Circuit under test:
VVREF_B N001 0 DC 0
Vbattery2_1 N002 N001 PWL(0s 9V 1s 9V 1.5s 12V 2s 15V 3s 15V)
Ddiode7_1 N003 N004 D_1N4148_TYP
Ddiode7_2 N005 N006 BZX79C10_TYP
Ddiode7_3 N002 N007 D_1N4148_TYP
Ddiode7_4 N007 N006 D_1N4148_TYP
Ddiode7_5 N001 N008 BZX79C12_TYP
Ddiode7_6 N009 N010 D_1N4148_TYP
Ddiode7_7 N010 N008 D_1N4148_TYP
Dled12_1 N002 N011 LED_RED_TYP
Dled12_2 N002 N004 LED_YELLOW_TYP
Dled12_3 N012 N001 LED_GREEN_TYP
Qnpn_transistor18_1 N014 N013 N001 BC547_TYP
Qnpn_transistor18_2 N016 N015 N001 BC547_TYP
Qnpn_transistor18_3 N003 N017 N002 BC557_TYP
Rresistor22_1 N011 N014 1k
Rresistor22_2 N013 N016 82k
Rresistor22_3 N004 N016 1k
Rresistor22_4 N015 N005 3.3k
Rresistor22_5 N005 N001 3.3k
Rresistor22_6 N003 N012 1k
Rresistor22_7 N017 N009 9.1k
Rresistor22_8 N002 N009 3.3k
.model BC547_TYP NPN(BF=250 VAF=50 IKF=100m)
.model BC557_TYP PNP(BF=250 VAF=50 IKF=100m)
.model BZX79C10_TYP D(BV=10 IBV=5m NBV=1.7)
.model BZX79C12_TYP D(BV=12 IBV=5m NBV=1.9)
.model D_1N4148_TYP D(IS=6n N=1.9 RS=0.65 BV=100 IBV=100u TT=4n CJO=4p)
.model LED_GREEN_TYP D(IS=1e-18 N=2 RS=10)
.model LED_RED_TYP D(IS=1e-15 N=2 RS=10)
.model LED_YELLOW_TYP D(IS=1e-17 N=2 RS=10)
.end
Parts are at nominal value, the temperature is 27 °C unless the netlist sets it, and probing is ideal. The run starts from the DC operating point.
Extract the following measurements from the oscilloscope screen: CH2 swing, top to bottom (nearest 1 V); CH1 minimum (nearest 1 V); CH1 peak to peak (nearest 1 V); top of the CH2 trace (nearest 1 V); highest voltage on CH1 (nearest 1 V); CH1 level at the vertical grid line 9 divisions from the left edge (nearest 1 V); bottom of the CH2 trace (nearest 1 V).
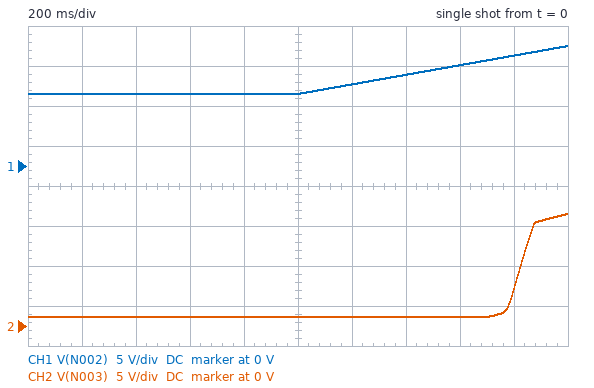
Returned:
13 V
9 V
6 V
14 V
15 V
14 V
1 V
